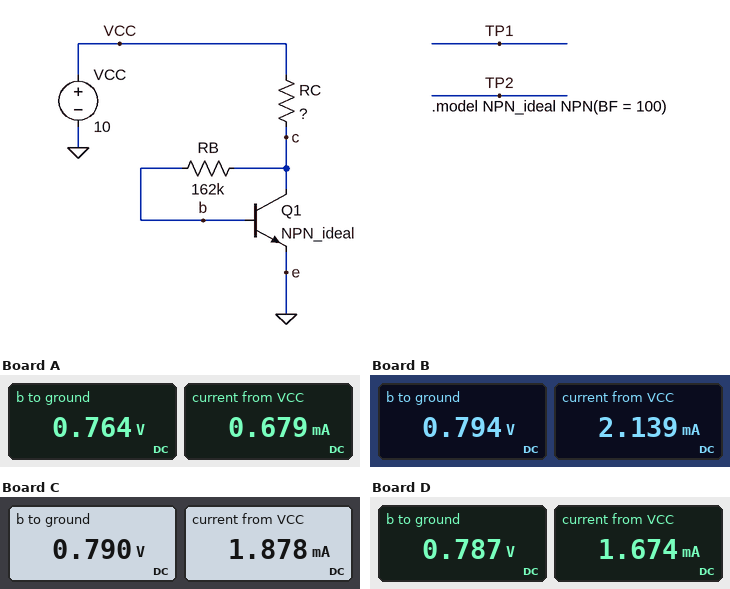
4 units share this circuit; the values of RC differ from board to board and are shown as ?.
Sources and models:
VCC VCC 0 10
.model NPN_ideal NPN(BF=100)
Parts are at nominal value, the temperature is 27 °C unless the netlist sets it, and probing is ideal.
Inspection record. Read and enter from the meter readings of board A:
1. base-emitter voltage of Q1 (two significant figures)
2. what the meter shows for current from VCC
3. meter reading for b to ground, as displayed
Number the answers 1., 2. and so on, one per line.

1. 760 mV
2. 0.679 mA
3. 0.764 V
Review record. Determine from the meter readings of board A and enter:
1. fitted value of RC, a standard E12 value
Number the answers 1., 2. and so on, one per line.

1. 12 kΩ
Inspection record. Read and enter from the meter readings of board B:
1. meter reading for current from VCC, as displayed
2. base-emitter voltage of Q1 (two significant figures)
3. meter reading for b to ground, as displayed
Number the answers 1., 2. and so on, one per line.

1. 2.139 mA
2. 790 mV
3. 0.794 V
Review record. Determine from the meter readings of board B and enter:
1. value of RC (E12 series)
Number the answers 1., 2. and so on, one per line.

1. 2.7 kΩ
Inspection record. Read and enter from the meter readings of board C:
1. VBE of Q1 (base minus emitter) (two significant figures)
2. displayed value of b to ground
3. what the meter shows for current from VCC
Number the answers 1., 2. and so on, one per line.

1. 790 mV
2. 0.790 V
3. 1.878 mA
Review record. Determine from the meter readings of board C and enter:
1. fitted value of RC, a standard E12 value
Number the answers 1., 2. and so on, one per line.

1. 3.3 kΩ
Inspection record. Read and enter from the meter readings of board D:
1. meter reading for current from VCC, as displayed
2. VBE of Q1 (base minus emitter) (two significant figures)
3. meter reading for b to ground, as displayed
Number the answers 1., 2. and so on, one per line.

1. 1.674 mA
2. 790 mV
3. 0.787 V
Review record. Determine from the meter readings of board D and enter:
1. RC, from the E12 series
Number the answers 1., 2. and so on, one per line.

1. 3.9 kΩ
